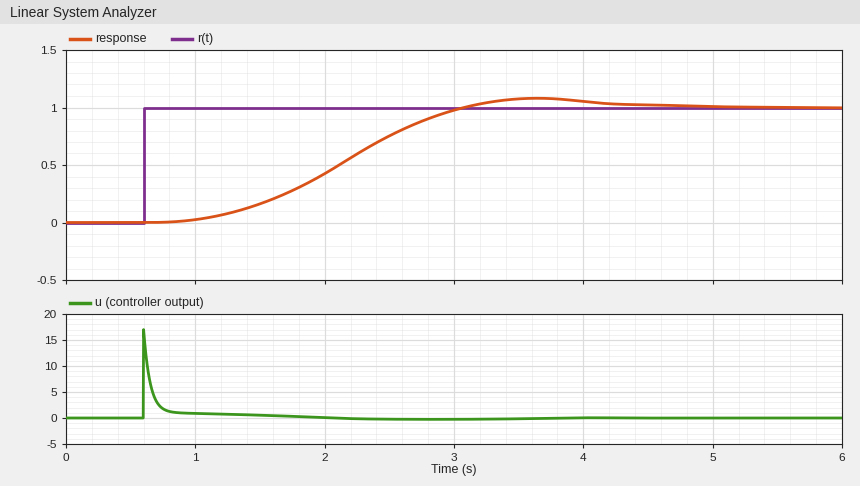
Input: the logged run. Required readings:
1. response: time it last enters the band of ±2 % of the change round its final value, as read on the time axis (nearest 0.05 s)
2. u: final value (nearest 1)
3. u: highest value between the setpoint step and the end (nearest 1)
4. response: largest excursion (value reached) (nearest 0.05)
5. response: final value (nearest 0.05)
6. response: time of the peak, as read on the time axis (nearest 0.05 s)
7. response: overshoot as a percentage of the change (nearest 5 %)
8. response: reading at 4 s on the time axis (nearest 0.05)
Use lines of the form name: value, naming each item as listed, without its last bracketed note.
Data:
response: time it last enters the band of ±2 % of the change round its final value, as read on the time axis: 4.65 s
u: final value: 0
u: highest value between the setpoint step and the end: 17
response: largest excursion (value reached): 1.10
response: final value: 1.00
response: time of the peak, as read on the time axis: 3.65 s
response: overshoot as a percentage of the change: 10 %
response: reading at 4 s on the time axis: 1.05
